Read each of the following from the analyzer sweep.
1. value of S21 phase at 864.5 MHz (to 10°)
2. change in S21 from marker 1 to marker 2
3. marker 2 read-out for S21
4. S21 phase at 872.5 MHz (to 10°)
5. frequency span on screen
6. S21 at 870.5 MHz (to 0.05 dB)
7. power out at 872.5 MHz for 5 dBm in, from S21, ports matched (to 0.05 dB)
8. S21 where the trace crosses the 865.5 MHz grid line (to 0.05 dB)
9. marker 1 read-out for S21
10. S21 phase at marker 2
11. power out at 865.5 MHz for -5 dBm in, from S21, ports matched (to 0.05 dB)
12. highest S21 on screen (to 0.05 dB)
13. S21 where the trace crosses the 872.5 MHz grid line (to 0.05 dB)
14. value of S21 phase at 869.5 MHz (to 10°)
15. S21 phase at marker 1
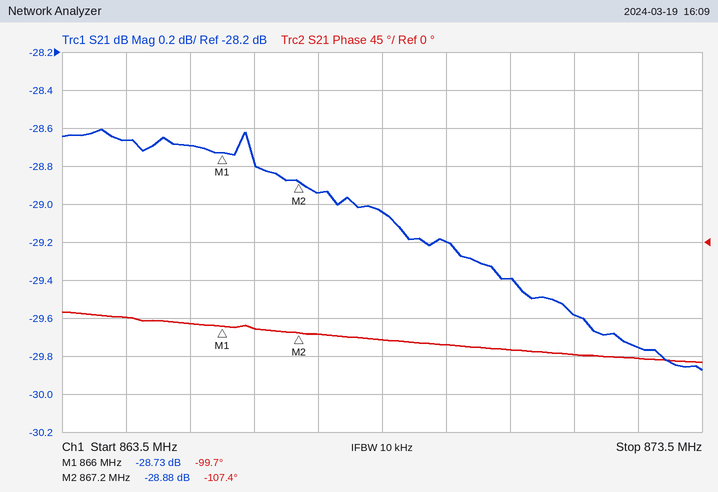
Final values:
-90°
-0.15 dB
-28.88 dB
-140°
10 MHz
-29.40 dB
-24.75 dBm
-28.70 dB
-28.73 dB
-107.4°
-33.70 dBm
-28.60 dB
-29.75 dB
-120°
-99.7°
